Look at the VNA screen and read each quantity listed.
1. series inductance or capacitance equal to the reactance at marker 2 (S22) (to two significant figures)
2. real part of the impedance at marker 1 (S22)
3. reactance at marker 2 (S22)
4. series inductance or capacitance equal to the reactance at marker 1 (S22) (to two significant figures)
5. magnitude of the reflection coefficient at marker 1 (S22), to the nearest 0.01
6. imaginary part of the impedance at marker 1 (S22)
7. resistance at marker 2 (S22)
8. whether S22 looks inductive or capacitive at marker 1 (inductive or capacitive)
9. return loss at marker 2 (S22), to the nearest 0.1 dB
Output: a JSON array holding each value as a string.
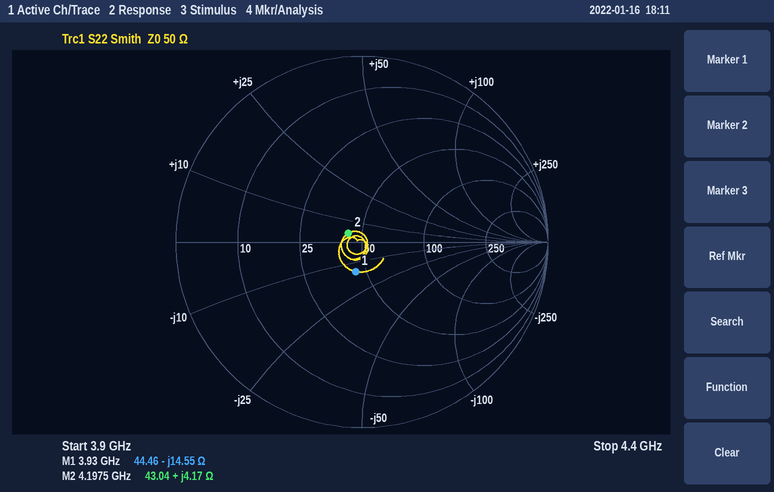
["160 pH", "44.46 Ω", "+4.17 Ω", "2.8 pF", "0.16", "-14.55 Ω", "43.04 Ω", "capacitive", "21.2 dB"]
